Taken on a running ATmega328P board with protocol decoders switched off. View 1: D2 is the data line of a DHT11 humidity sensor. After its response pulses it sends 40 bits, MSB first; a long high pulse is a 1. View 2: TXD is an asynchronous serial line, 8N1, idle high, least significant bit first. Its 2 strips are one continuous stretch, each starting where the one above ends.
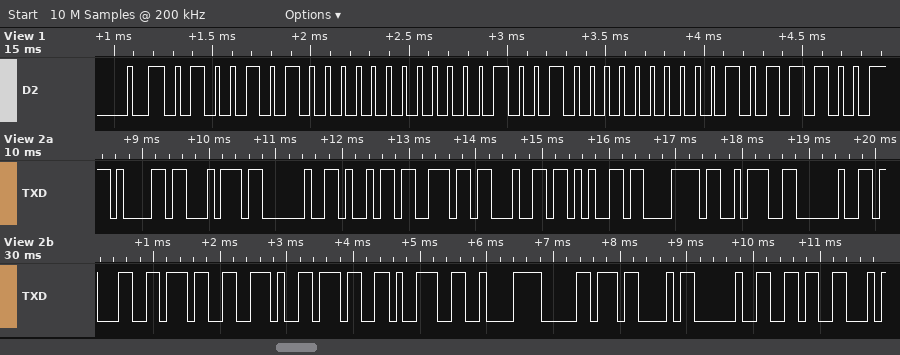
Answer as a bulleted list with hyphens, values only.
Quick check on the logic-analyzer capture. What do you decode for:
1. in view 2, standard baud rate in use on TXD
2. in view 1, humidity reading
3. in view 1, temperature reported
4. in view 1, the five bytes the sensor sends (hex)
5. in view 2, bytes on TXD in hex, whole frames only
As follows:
- 9600 baud
- 74 %
- 18.0 °C
- 4A 00 12 00 5C
- 0x61 0x74 0x20 0x69 0x6E 0x64 0x65 0x78 0x3A 0x20 0x31 0x37 0x2E 0x37 0x39 0xC2 0xB0 0x43 0x20 0x36
